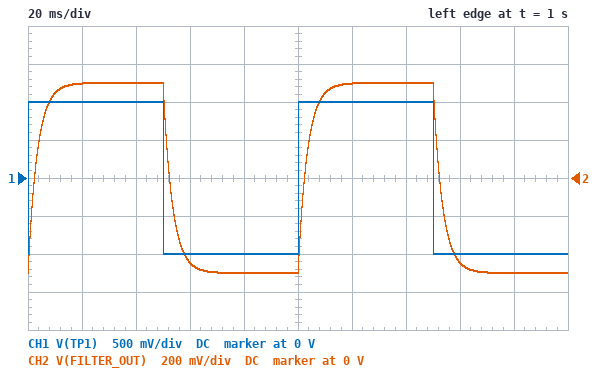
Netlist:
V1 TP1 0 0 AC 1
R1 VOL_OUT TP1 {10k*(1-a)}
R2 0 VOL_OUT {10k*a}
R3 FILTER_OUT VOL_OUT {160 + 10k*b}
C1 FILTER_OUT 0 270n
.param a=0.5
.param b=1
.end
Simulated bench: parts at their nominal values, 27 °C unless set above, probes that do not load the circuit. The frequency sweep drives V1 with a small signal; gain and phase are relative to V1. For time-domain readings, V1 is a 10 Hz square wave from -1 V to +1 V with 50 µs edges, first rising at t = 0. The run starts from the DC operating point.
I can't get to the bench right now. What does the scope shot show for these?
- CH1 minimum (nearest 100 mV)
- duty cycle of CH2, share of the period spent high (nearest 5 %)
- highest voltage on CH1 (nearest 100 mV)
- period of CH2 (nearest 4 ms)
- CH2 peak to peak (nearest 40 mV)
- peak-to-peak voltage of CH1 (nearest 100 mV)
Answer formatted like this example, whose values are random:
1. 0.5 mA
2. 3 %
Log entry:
1. -1.0 V
2. 50 %
3. 1.0 V
4. 100 ms
5. 1.00 V
6. 2.0 V
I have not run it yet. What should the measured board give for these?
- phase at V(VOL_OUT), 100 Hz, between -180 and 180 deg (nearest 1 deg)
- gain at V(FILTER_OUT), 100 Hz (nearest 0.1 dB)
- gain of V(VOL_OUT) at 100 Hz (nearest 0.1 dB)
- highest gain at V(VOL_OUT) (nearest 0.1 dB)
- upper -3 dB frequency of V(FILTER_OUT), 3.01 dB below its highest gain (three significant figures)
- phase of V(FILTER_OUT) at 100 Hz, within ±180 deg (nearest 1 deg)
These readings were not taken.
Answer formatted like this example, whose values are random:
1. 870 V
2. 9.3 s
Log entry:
1. -5 deg
2. -13.5 dB
3. -7.5 dB
4. -6.0 dB
5. 46.6 Hz
6. -65 deg
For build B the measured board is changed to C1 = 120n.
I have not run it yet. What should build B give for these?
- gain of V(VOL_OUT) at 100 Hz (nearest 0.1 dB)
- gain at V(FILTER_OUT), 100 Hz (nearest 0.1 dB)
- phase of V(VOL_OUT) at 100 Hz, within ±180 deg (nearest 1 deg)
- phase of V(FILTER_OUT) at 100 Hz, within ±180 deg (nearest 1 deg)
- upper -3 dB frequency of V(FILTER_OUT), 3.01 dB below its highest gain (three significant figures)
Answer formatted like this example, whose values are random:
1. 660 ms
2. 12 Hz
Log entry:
1. -6.8 dB
2. -8.8 dB
3. -6 deg
4. -44 deg
5. 105 Hz
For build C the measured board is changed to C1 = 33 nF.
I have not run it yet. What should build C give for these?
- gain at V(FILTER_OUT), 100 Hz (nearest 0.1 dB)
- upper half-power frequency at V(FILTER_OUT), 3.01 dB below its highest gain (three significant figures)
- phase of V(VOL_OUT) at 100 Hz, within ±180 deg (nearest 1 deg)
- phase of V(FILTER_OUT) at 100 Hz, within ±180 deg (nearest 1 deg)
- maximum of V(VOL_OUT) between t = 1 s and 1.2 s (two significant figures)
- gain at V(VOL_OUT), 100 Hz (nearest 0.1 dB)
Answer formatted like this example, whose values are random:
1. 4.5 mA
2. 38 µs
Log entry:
1. -6.3 dB
2. 381 Hz
3. -3 deg
4. -15 deg
5. 500 mV
6. -6.1 dB
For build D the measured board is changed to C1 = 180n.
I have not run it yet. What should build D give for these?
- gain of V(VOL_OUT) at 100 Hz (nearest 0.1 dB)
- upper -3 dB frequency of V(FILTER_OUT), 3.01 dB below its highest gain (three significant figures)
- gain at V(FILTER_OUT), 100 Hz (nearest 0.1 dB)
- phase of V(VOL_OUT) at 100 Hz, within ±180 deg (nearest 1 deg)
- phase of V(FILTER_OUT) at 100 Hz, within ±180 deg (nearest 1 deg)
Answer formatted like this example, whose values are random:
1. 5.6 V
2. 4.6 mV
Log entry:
1. -7.2 dB
2. 69.8 Hz
3. -10.9 dB
4. -6 deg
5. -55 deg
